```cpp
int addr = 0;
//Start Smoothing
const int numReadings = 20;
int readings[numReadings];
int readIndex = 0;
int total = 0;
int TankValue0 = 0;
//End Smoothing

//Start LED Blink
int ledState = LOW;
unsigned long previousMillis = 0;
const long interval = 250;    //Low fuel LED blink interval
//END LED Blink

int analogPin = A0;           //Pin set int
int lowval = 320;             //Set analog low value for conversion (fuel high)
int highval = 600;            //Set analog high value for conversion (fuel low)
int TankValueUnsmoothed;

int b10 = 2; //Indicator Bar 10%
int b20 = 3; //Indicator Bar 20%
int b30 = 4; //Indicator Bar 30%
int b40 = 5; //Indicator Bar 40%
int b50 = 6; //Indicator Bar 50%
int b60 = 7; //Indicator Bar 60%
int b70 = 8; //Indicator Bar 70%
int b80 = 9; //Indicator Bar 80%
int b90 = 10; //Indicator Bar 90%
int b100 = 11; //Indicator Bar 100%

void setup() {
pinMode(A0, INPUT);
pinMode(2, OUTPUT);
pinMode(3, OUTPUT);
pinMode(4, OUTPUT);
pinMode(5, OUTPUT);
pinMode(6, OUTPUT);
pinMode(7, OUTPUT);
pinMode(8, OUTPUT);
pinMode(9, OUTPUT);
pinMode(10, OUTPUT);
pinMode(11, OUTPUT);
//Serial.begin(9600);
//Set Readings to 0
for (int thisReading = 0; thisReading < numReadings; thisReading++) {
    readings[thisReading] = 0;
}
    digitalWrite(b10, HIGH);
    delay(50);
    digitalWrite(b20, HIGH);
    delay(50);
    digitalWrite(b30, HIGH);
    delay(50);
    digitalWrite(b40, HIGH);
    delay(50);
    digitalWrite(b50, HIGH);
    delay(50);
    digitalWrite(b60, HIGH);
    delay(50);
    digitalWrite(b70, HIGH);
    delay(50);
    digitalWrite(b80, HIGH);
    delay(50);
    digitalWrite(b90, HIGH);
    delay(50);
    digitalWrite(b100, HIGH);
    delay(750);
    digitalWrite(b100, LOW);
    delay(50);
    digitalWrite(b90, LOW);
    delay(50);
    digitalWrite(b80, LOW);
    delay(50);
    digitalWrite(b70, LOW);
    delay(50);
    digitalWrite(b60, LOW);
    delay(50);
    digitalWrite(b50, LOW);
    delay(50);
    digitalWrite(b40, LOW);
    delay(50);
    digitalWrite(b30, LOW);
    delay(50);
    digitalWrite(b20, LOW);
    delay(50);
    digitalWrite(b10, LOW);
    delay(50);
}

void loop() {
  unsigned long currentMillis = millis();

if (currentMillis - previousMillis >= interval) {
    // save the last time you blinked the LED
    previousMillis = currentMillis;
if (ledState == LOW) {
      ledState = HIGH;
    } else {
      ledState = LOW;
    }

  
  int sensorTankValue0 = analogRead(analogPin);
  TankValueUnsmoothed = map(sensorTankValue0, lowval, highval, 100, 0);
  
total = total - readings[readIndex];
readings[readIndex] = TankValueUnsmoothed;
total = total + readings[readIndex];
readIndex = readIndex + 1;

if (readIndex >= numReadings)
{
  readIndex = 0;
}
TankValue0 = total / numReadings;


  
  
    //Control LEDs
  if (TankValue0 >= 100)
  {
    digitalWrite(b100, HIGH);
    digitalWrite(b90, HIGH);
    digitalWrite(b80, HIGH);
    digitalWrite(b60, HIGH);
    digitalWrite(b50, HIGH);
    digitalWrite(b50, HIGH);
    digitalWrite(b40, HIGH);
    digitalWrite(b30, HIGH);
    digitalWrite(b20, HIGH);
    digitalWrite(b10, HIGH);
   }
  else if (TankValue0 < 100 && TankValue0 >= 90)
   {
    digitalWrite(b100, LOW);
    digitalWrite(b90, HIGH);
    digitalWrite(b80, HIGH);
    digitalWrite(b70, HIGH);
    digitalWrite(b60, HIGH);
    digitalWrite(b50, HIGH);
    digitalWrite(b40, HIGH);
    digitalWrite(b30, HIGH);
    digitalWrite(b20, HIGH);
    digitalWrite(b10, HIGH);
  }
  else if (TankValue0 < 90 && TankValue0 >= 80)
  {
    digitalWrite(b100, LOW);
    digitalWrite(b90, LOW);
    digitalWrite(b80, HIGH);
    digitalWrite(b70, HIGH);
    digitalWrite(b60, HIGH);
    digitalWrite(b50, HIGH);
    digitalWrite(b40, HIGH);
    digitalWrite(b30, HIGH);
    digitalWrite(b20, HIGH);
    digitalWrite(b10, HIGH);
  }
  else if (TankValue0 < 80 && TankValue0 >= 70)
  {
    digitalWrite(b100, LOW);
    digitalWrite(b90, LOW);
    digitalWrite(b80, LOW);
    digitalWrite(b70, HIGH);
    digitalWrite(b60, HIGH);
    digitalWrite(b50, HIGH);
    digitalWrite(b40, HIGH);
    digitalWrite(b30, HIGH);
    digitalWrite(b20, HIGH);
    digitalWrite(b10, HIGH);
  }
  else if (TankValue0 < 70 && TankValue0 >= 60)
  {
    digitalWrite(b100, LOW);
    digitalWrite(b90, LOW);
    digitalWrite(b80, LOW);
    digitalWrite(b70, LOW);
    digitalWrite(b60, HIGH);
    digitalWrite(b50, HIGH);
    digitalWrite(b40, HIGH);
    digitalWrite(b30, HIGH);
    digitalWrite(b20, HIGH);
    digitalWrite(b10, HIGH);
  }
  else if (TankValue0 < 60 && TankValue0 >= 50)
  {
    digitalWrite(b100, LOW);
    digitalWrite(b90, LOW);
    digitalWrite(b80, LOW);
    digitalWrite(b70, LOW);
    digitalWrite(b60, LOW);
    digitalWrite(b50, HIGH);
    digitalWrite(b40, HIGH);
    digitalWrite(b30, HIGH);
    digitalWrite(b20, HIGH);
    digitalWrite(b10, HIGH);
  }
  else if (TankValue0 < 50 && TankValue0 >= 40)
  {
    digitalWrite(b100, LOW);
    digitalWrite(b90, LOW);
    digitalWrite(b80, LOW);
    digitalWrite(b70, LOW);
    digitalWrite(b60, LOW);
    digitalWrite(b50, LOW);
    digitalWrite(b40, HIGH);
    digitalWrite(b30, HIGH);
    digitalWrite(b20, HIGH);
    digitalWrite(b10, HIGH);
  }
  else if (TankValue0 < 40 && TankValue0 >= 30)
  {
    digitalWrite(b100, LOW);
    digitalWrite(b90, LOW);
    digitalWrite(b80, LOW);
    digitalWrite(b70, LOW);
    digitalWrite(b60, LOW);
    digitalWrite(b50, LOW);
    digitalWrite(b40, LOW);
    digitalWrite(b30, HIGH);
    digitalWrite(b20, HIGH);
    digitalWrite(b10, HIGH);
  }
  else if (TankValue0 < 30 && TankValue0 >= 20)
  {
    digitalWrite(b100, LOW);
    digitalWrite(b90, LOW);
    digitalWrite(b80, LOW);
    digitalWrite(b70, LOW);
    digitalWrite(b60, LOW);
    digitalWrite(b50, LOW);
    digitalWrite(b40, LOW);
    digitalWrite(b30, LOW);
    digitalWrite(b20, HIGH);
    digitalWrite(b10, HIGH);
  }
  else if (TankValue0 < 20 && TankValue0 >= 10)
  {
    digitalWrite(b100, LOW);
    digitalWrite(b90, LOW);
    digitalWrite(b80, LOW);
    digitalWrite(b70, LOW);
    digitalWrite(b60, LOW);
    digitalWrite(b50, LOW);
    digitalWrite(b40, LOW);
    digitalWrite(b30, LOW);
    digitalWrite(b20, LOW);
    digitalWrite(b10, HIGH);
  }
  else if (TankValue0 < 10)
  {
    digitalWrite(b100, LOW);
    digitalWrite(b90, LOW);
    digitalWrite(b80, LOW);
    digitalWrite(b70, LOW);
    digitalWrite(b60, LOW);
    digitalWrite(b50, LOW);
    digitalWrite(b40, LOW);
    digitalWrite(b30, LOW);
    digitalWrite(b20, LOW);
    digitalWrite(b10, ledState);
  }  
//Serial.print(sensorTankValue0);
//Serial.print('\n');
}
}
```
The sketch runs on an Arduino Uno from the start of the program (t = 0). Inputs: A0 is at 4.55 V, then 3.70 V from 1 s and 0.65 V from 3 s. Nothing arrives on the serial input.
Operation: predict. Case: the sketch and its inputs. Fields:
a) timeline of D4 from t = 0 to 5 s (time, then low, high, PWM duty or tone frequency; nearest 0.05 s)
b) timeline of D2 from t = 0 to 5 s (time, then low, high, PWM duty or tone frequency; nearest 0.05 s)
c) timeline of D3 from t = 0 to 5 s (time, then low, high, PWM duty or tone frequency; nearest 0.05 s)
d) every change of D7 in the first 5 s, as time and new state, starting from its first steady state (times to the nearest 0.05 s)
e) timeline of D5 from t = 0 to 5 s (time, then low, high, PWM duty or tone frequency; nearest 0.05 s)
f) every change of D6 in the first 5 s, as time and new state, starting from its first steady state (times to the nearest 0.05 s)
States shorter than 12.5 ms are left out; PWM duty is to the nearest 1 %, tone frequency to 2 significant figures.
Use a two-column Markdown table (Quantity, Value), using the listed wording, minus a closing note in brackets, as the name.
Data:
| Quantity | Value |
|---|---|
| timeline of D4 from t = 0 to 5 s | 0 s low; 0.1 s high; 1.55 s low; 4.45 s high |
| timeline of D2 from t = 0 to 5 s | 0 s high; 1.65 s low; 1.7 s high; 1.95 s low; 2.2 s high; 2.45 s low; 2.7 s high; 2.95 s low; 3.2 s high; 3.45 s low; 3.7 s high |
| timeline of D3 from t = 0 to 5 s | 0 s low; 0.05 s high; 1.6 s low; 4.2 s high |
| every change of D7 in the first 5 s, as time and new state, starting from its first steady state | 0 s low; 0.25 s high; 1.4 s low |
| timeline of D5 from t = 0 to 5 s | 0 s low; 0.15 s high; 1.5 s low; 4.7 s high |
| every change of D6 in the first 5 s, as time and new state, starting from its first steady state | 0 s low; 0.2 s high; 1.45 s low |
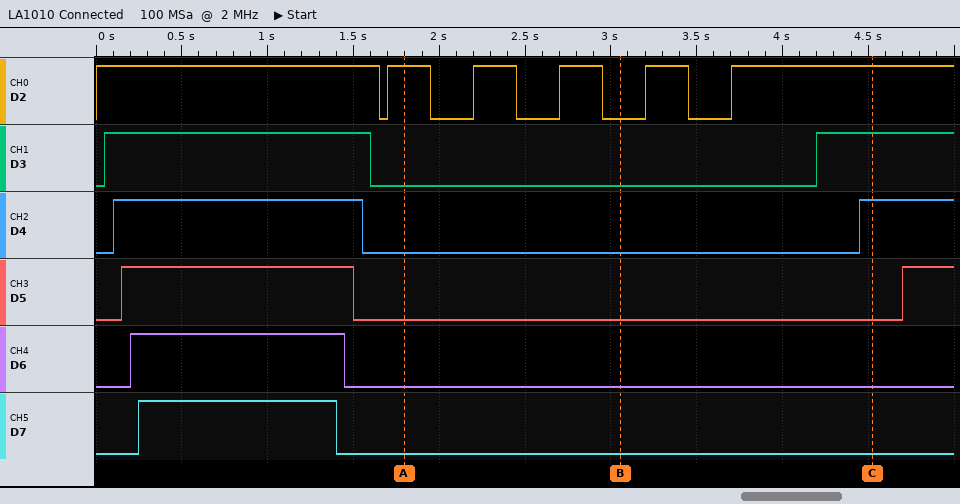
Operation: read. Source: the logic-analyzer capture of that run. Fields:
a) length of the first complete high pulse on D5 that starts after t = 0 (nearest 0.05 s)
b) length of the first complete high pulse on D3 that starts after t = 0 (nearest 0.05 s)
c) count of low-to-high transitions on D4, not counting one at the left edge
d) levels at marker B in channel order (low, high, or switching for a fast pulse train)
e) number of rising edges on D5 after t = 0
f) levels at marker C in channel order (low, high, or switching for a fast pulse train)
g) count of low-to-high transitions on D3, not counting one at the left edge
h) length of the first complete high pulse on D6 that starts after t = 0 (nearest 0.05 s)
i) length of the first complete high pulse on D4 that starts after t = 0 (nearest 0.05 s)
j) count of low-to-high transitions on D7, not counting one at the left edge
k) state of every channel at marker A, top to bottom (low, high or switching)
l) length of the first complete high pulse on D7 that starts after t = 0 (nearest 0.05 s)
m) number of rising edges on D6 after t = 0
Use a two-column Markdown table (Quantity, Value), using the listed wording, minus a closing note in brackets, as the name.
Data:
| Quantity | Value |
|---|---|
| length of the first complete high pulse on D5 that starts after t = 0 | 1.35 s |
| length of the first complete high pulse on D3 that starts after t = 0 | 1.55 s |
| count of low-to-high transitions on D4, not counting one at the left edge | 2 |
| levels at marker B in channel order | D2 low, D3 low, D4 low, D5 low, D6 low, D7 low |
| number of rising edges on D5 after t = 0 | 2 |
| levels at marker C in channel order | D2 high, D3 high, D4 high, D5 low, D6 low, D7 low |
| count of low-to-high transitions on D3, not counting one at the left edge | 2 |
| length of the first complete high pulse on D6 that starts after t = 0 | 1.25 s |
| length of the first complete high pulse on D4 that starts after t = 0 | 1.45 s |
| count of low-to-high transitions on D7, not counting one at the left edge | 1 |
| state of every channel at marker A, top to bottom | D2 high, D3 low, D4 low, D5 low, D6 low, D7 low |
| length of the first complete high pulse on D7 that starts after t = 0 | 1.15 s |
| number of rising edges on D6 after t = 0 | 1 |
